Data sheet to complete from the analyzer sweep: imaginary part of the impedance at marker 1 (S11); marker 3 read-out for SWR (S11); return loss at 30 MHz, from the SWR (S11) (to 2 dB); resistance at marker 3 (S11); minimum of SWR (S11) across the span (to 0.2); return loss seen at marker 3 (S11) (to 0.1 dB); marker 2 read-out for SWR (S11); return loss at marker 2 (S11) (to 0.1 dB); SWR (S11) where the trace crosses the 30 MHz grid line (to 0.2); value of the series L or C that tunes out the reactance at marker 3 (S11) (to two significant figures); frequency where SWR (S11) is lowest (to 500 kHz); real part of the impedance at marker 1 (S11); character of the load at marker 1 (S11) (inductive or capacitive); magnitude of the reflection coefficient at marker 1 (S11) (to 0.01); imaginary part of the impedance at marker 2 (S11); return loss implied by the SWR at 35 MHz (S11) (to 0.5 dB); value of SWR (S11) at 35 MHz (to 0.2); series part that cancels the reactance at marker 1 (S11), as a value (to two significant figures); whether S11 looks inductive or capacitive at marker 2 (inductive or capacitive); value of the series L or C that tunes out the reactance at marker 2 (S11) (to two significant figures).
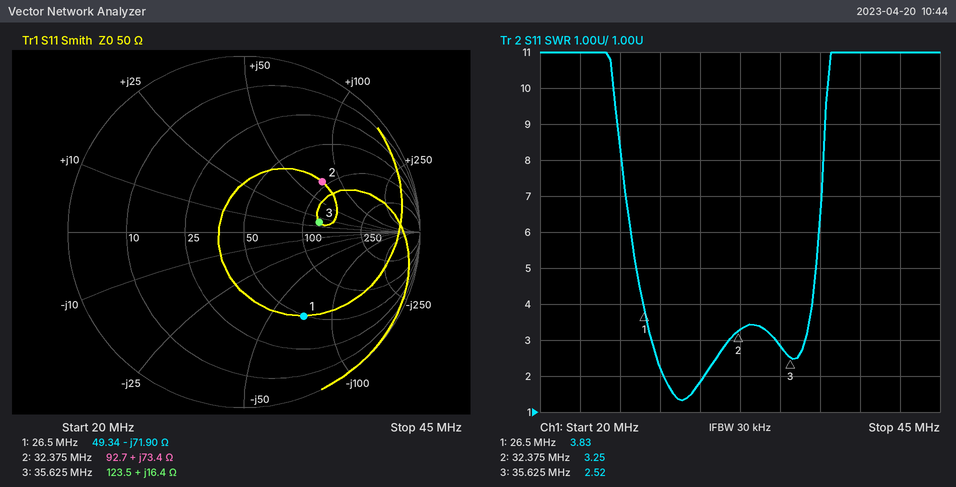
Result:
-71.90 Ω
2.52
10 dB
123.5 Ω
1.4
7.3 dB
3.25
5.5 dB
1.8
270 pF
29.0 MHz
49.34 Ω
capacitive
0.59
+73.4 Ω
6.5 dB
2.8
430 nH
inductive
67 pF
